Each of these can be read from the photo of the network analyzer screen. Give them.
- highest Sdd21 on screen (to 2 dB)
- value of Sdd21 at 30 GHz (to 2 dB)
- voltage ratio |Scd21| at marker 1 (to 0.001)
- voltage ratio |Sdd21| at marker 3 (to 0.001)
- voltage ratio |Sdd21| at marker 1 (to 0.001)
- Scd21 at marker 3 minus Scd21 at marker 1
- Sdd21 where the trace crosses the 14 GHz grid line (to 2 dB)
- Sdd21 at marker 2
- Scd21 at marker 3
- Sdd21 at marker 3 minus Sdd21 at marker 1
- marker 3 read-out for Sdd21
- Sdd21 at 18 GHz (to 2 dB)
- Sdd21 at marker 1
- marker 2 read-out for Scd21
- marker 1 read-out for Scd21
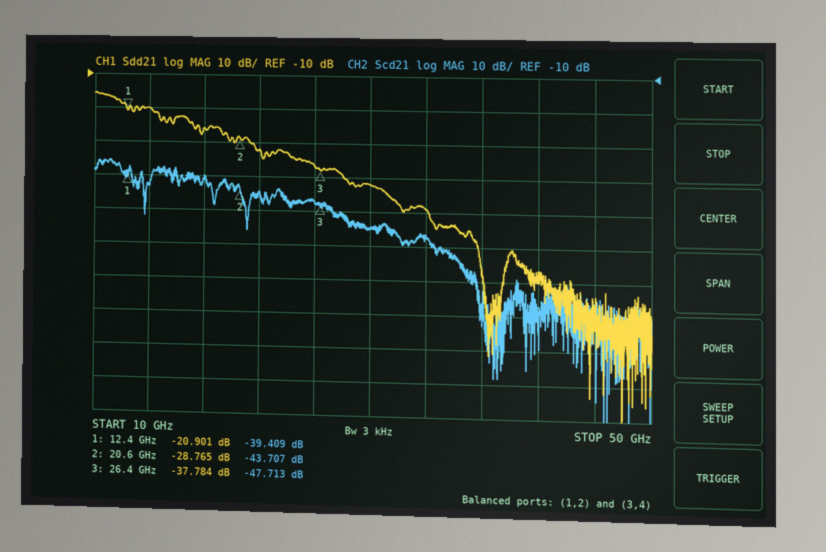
-16 dB
-42 dB
0.011
0.013
0.090
-8.304 dB
-20 dB
-28.765 dB
-47.713 dB
-16.883 dB
-37.784 dB
-26 dB
-20.901 dB
-43.707 dB
-39.409 dB
